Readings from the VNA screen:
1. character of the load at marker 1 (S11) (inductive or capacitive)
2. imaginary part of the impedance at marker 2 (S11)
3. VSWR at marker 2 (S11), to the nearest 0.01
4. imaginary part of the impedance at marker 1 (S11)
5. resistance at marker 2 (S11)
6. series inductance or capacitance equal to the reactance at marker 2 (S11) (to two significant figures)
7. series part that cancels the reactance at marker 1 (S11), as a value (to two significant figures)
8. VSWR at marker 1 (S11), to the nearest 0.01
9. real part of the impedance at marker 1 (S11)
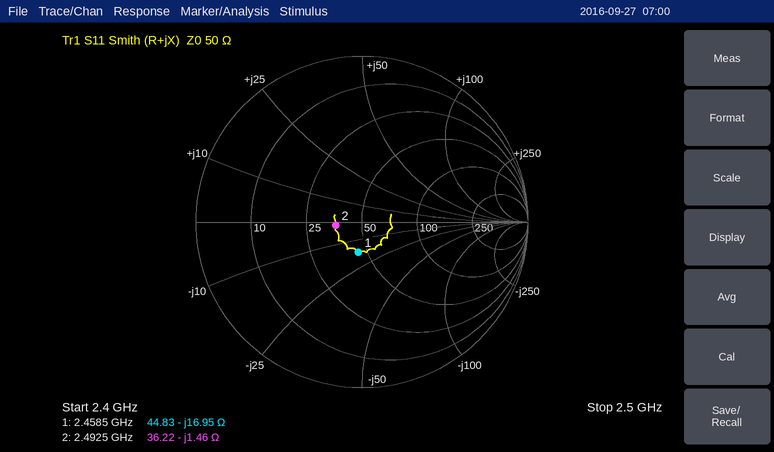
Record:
capacitive
-1.46 Ω
1.38
-16.95 Ω
36.22 Ω
44 pF
1.1 nH
1.45
44.83 Ω
